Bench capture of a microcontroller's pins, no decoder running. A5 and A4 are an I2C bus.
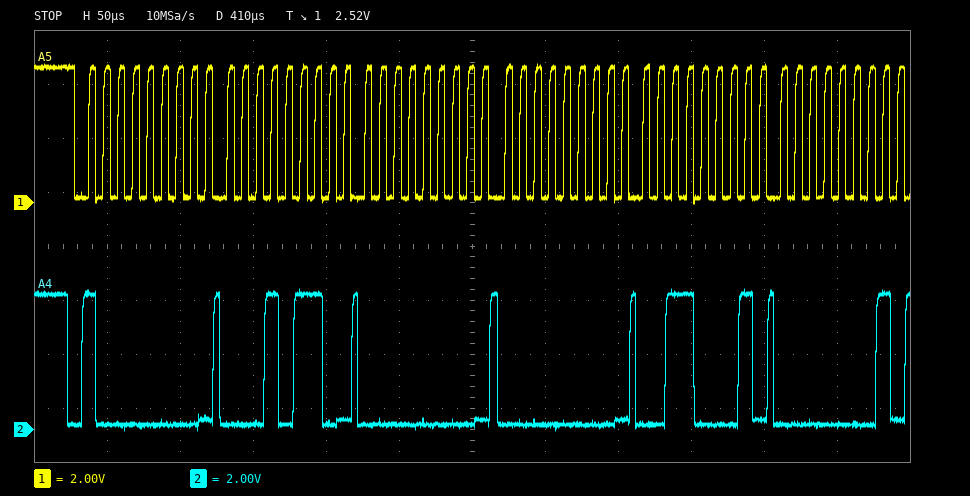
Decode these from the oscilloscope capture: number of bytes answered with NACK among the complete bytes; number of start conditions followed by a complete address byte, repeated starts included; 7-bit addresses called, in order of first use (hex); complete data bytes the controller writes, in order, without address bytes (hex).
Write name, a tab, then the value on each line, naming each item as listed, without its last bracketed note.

number of bytes answered with NACK among the complete bytes	0
number of start conditions followed by a complete address byte, repeated starts included	1
7-bit addresses called, in order of first use	0x40
complete data bytes the controller writes, in order, without address bytes	16 00 00 31 01
